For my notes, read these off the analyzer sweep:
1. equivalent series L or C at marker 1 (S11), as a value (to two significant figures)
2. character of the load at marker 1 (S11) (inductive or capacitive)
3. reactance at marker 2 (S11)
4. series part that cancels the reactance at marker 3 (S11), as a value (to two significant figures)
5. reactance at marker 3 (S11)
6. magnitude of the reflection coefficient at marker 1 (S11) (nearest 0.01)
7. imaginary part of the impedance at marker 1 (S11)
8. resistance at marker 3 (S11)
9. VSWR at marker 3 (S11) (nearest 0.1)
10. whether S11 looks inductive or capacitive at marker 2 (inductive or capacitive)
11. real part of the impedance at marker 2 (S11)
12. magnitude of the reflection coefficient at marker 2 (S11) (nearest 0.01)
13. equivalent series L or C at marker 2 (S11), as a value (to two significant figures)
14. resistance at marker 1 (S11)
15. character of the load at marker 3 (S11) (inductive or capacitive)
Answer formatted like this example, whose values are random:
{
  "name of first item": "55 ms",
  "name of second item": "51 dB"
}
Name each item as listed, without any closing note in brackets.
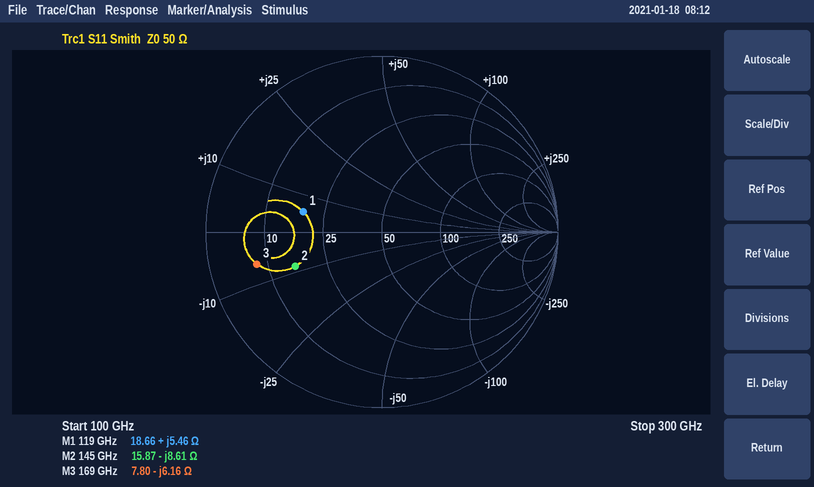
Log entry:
{
  "equivalent series L or C at marker 1 (S11), as a value": "7.3 pH",
  "character of the load at marker 1 (S11)": "inductive",
  "reactance at marker 2": "-8.61 Ω",
  "series part that cancels the reactance at marker 3 (S11), as a value": "5.8 pH",
  "reactance at marker 3": "-6.16 Ω",
  "magnitude of the reflection coefficient at marker 1 (S11)": "0.46",
  "imaginary part of the impedance at marker 1": "+5.46 Ω",
  "resistance at marker 3": "7.80 Ω",
  "VSWR at marker 3 (S11)": "6.5",
  "whether S11 looks inductive or capacitive at marker 2": "capacitive",
  "real part of the impedance at marker 2": "15.87 Ω",
  "magnitude of the reflection coefficient at marker 2 (S11)": "0.53",
  "equivalent series L or C at marker 2 (S11), as a value": "130 fF",
  "resistance at marker 1": "18.66 Ω",
  "character of the load at marker 3 (S11)": "capacitive"
}
